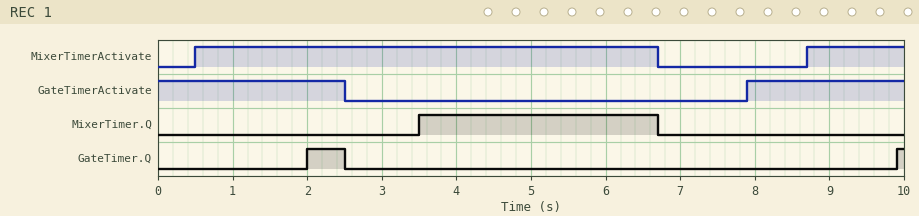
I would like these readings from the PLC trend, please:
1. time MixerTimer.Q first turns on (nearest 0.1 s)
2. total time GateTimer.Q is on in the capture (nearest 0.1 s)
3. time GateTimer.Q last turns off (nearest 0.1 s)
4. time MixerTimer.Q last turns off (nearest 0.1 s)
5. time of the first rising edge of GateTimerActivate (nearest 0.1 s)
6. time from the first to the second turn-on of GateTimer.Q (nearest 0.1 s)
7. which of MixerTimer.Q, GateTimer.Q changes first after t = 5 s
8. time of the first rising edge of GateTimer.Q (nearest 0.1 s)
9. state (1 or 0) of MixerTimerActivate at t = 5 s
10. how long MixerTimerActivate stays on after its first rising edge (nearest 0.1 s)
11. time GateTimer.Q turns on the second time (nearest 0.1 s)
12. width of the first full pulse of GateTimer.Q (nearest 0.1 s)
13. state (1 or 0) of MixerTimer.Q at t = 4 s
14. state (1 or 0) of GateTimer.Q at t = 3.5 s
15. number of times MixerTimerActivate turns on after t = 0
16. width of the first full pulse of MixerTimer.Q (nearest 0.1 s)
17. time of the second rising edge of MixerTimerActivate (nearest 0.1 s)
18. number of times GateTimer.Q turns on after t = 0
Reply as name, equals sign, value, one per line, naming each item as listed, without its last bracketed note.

time MixerTimer.Q first turns on = 3.5 s
total time GateTimer.Q is on in the capture = 0.6 s
time GateTimer.Q last turns off = 2.5 s
time MixerTimer.Q last turns off = 6.7 s
time of the first rising edge of GateTimerActivate = 7.9 s
time from the first to the second turn-on of GateTimer.Q = 7.9 s
which of MixerTimer.Q, GateTimer.Q changes first after t = 5 s = MixerTimer.Q
time of the first rising edge of GateTimer.Q = 2.0 s
state (1 or 0) of MixerTimerActivate at t = 5 s = 1
how long MixerTimerActivate stays on after its first rising edge = 6.2 s
time GateTimer.Q turns on the second time = 9.9 s
width of the first full pulse of GateTimer.Q = 0.5 s
state (1 or 0) of MixerTimer.Q at t = 4 s = 1
state (1 or 0) of GateTimer.Q at t = 3.5 s = 0
number of times MixerTimerActivate turns on after t = 0 = 2
width of the first full pulse of MixerTimer.Q = 3.2 s
time of the second rising edge of MixerTimerActivate = 8.7 s
number of times GateTimer.Q turns on after t = 0 = 2
